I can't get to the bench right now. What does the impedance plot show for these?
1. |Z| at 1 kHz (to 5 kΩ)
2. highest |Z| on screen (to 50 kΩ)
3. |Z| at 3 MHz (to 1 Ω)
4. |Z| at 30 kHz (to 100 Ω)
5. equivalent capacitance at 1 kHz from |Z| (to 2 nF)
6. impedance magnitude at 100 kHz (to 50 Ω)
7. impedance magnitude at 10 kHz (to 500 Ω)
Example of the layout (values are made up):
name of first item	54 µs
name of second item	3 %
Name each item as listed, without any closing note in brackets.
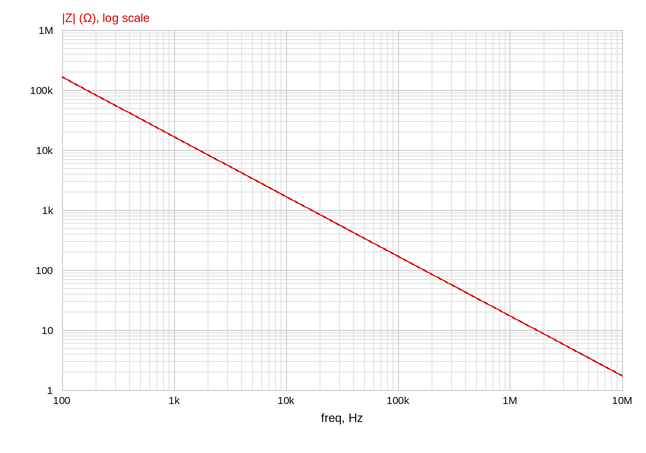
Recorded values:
|Z| at 1 kHz	15 kΩ
highest |Z| on screen	150 kΩ
|Z| at 3 MHz	6 Ω
|Z| at 30 kHz	600 Ω
equivalent capacitance at 1 kHz from |Z|	10 nF
impedance magnitude at 100 kHz	150 Ω
impedance magnitude at 10 kHz	1.5 kΩ
